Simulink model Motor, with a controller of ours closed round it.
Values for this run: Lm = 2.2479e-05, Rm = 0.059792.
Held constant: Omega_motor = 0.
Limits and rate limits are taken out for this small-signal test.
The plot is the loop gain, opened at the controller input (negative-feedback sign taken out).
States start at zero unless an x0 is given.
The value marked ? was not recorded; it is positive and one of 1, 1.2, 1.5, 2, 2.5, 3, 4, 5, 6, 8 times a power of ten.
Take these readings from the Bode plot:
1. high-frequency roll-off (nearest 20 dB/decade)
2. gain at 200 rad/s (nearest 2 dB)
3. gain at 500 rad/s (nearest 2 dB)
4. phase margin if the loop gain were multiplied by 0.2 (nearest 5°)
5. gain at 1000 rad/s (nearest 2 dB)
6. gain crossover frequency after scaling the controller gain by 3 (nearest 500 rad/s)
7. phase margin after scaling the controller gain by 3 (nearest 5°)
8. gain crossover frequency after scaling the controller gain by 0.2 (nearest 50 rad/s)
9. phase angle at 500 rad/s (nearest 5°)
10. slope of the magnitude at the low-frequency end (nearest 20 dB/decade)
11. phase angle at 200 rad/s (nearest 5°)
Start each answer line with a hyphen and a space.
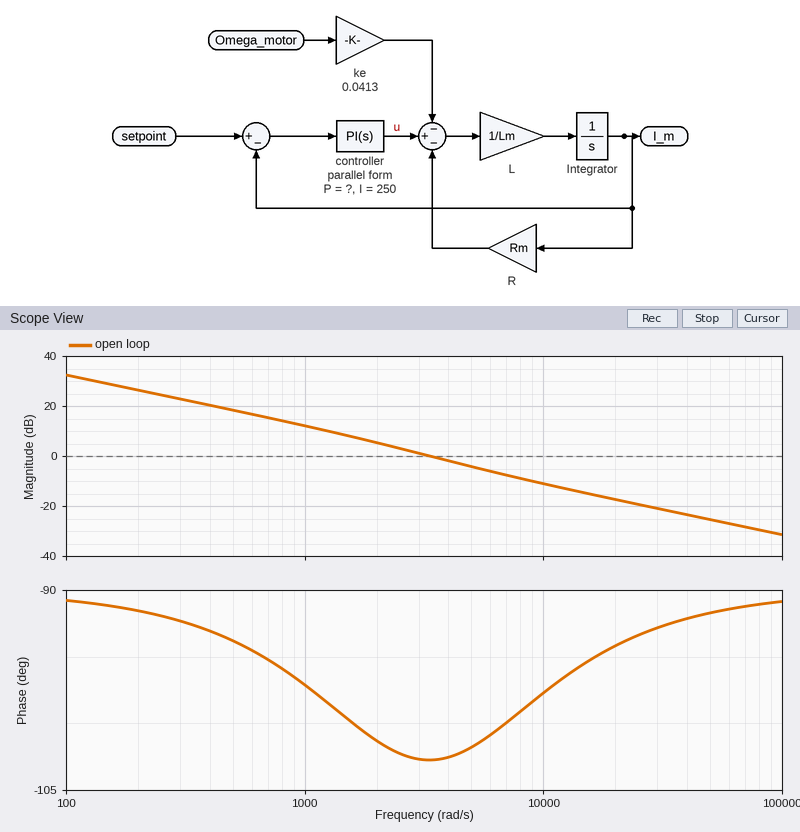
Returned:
- -20 dB/decade
- 26 dB
- 18 dB
- 85°
- 12 dB
- 8500 rad/s
- 80°
- 800 rad/s
- -95°
- -20 dB/decade
- -90°
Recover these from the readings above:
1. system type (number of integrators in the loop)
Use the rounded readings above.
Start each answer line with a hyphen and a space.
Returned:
- 1
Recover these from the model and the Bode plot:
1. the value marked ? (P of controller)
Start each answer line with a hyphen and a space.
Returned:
- 0.06
